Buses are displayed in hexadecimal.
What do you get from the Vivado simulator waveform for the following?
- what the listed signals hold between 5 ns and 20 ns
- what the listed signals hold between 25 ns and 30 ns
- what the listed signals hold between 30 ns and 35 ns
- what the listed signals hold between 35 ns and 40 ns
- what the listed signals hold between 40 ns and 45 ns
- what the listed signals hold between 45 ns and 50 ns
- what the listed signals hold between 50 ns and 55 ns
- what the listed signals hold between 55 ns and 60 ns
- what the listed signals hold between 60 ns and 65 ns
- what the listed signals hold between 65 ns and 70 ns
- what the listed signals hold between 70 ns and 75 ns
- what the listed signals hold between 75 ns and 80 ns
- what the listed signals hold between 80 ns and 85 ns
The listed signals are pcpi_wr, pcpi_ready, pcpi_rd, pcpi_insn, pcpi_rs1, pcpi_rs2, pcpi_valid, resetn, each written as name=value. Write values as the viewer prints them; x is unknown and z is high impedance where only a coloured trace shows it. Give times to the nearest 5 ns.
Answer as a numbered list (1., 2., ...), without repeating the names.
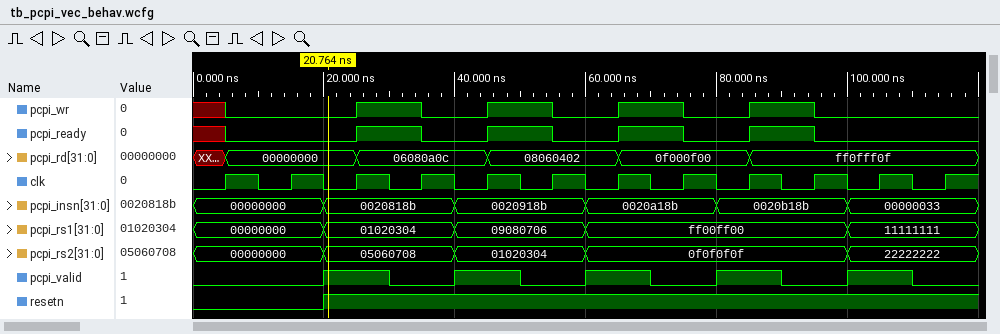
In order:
1. pcpi_wr=0, pcpi_ready=0, pcpi_rd=00000000, pcpi_insn=00000000, pcpi_rs1=00000000, pcpi_rs2=00000000, pcpi_valid=0, resetn=0
2. pcpi_wr=1, pcpi_ready=1, pcpi_rd=06080a0c, pcpi_insn=0020818b, pcpi_rs1=01020304, pcpi_rs2=05060708, pcpi_valid=1, resetn=1
3. pcpi_wr=1, pcpi_ready=1, pcpi_rd=06080a0c, pcpi_insn=0020818b, pcpi_rs1=01020304, pcpi_rs2=05060708, pcpi_valid=0, resetn=1
4. pcpi_wr=0, pcpi_ready=0, pcpi_rd=06080a0c, pcpi_insn=0020818b, pcpi_rs1=01020304, pcpi_rs2=05060708, pcpi_valid=0, resetn=1
5. pcpi_wr=0, pcpi_ready=0, pcpi_rd=06080a0c, pcpi_insn=0020918b, pcpi_rs1=09080706, pcpi_rs2=01020304, pcpi_valid=1, resetn=1
6. pcpi_wr=1, pcpi_ready=1, pcpi_rd=08060402, pcpi_insn=0020918b, pcpi_rs1=09080706, pcpi_rs2=01020304, pcpi_valid=1, resetn=1
7. pcpi_wr=1, pcpi_ready=1, pcpi_rd=08060402, pcpi_insn=0020918b, pcpi_rs1=09080706, pcpi_rs2=01020304, pcpi_valid=0, resetn=1
8. pcpi_wr=0, pcpi_ready=0, pcpi_rd=08060402, pcpi_insn=0020918b, pcpi_rs1=09080706, pcpi_rs2=01020304, pcpi_valid=0, resetn=1
9. pcpi_wr=0, pcpi_ready=0, pcpi_rd=08060402, pcpi_insn=0020a18b, pcpi_rs1=ff00ff00, pcpi_rs2=0f0f0f0f, pcpi_valid=1, resetn=1
10. pcpi_wr=1, pcpi_ready=1, pcpi_rd=0f000f00, pcpi_insn=0020a18b, pcpi_rs1=ff00ff00, pcpi_rs2=0f0f0f0f, pcpi_valid=1, resetn=1
11. pcpi_wr=1, pcpi_ready=1, pcpi_rd=0f000f00, pcpi_insn=0020a18b, pcpi_rs1=ff00ff00, pcpi_rs2=0f0f0f0f, pcpi_valid=0, resetn=1
12. pcpi_wr=0, pcpi_ready=0, pcpi_rd=0f000f00, pcpi_insn=0020a18b, pcpi_rs1=ff00ff00, pcpi_rs2=0f0f0f0f, pcpi_valid=0, resetn=1
13. pcpi_wr=0, pcpi_ready=0, pcpi_rd=0f000f00, pcpi_insn=0020b18b, pcpi_rs1=ff00ff00, pcpi_rs2=0f0f0f0f, pcpi_valid=1, resetn=1
